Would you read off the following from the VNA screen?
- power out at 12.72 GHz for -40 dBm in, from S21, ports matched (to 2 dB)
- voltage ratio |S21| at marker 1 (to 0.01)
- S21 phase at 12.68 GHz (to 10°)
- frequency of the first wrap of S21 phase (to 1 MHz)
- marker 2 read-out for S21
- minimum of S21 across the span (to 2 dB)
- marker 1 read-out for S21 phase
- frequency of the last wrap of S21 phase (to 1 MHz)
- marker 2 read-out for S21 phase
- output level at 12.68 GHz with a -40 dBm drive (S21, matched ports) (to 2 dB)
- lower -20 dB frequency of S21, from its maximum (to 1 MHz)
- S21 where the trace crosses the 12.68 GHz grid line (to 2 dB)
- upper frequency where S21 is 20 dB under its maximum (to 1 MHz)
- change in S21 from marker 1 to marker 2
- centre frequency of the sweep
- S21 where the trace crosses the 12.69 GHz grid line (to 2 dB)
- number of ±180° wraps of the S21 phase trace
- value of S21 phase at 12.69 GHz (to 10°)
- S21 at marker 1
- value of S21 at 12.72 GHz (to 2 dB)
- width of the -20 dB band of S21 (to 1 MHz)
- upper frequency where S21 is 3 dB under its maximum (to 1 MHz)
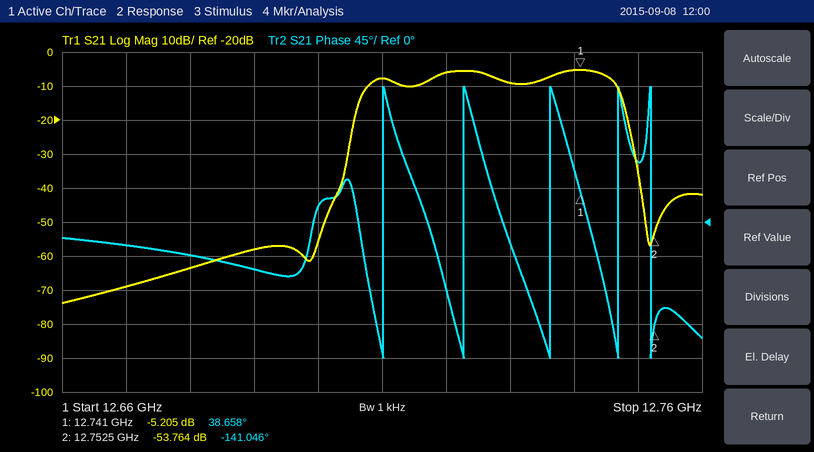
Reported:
-46 dBm
0.55
-40°
12.710 GHz
-53.764 dB
-74 dB
38.658°
12.752 GHz
-141.046°
-104 dBm
12.705 GHz
-64 dB
12.749 GHz
-48.559 dB
12.71 GHz
-58 dB
5
-60°
-5.205 dB
-6 dB
44 MHz
12.746 GHz
